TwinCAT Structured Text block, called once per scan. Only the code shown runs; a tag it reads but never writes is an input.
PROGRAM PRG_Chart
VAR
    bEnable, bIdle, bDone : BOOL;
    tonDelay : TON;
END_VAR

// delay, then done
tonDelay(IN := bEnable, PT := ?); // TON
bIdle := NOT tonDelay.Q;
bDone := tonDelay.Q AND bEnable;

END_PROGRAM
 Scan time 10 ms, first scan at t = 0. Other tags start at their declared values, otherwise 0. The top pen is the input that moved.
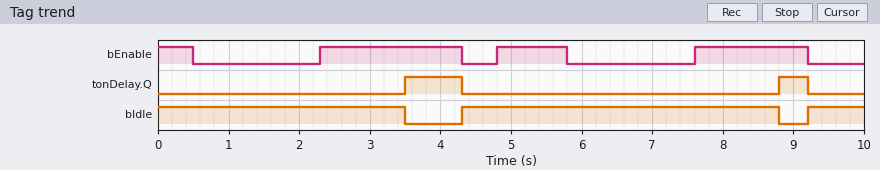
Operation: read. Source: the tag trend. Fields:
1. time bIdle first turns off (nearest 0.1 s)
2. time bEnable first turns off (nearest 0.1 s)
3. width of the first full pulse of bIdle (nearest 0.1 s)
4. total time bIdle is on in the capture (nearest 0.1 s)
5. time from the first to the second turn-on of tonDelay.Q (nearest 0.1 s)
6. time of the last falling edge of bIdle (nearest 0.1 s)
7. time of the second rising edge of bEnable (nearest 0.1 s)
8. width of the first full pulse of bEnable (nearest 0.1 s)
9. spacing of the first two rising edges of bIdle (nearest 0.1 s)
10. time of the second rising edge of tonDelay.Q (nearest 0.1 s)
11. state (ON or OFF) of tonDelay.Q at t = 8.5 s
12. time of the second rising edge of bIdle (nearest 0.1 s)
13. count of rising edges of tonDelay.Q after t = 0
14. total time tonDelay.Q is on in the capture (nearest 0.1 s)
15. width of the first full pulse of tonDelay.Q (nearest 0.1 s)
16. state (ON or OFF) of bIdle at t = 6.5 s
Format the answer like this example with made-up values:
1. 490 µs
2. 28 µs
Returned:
1. 3.5 s
2. 0.5 s
3. 4.5 s
4. 8.8 s
5. 5.3 s
6. 8.8 s
7. 4.8 s
8. 2.0 s
9. 4.9 s
10. 8.8 s
11. OFF
12. 9.2 s
13. 2
14. 1.2 s
15. 0.8 s
16. ON
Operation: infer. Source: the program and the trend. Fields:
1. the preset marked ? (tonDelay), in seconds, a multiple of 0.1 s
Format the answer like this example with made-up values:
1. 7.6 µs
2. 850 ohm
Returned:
1. 1.2 s
